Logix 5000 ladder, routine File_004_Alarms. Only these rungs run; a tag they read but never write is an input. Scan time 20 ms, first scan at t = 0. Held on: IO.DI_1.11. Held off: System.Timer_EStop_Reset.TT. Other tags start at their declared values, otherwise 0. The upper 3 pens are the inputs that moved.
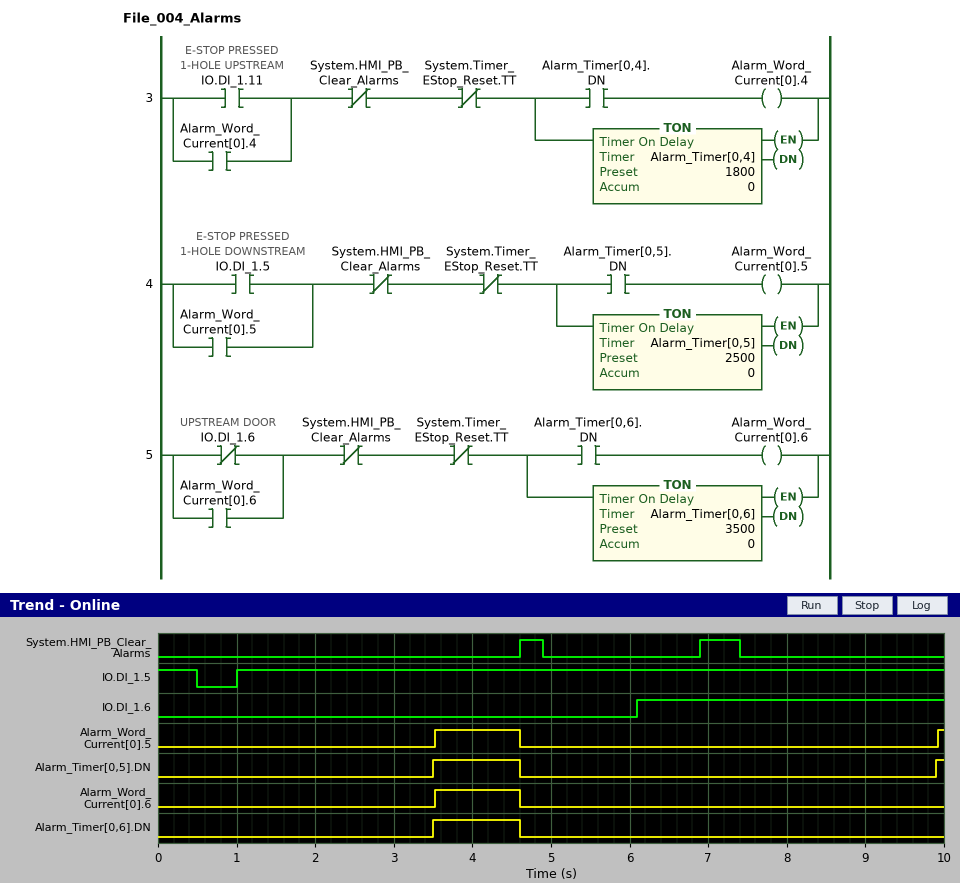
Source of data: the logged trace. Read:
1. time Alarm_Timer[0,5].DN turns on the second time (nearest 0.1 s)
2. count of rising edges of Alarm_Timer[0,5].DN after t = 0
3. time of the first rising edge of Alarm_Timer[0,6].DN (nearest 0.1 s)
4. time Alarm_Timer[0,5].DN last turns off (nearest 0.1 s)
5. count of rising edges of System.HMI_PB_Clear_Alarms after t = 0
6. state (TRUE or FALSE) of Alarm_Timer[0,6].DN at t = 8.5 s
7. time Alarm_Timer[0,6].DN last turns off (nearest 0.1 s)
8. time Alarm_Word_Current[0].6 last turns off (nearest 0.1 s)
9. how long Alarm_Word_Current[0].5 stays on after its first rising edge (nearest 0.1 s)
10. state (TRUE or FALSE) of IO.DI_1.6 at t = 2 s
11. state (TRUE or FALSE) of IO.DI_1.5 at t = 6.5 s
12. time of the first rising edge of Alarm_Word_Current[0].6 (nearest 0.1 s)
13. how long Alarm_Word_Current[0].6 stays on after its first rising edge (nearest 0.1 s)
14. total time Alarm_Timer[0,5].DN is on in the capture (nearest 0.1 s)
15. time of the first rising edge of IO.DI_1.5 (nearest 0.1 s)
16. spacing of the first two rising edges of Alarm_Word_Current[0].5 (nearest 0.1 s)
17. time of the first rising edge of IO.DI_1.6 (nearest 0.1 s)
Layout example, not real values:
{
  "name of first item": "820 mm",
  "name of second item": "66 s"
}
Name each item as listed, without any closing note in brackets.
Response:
{
  "time Alarm_Timer[0,5].DN turns on the second time": "9.9 s",
  "count of rising edges of Alarm_Timer[0,5].DN after t = 0": "2",
  "time of the first rising edge of Alarm_Timer[0,6].DN": "3.5 s",
  "time Alarm_Timer[0,5].DN last turns off": "4.6 s",
  "count of rising edges of System.HMI_PB_Clear_Alarms after t = 0": "2",
  "state (TRUE or FALSE) of Alarm_Timer[0,6].DN at t = 8.5 s": "FALSE",
  "time Alarm_Timer[0,6].DN last turns off": "4.6 s",
  "time Alarm_Word_Current[0].6 last turns off": "4.6 s",
  "how long Alarm_Word_Current[0].5 stays on after its first rising edge": "1.1 s",
  "state (TRUE or FALSE) of IO.DI_1.6 at t = 2 s": "FALSE",
  "state (TRUE or FALSE) of IO.DI_1.5 at t = 6.5 s": "TRUE",
  "time of the first rising edge of Alarm_Word_Current[0].6": "3.5 s",
  "how long Alarm_Word_Current[0].6 stays on after its first rising edge": "1.1 s",
  "total time Alarm_Timer[0,5].DN is on in the capture": "1.2 s",
  "time of the first rising edge of IO.DI_1.5": "1.0 s",
  "spacing of the first two rising edges of Alarm_Word_Current[0].5": "6.4 s",
  "time of the first rising edge of IO.DI_1.6": "6.1 s"
}
